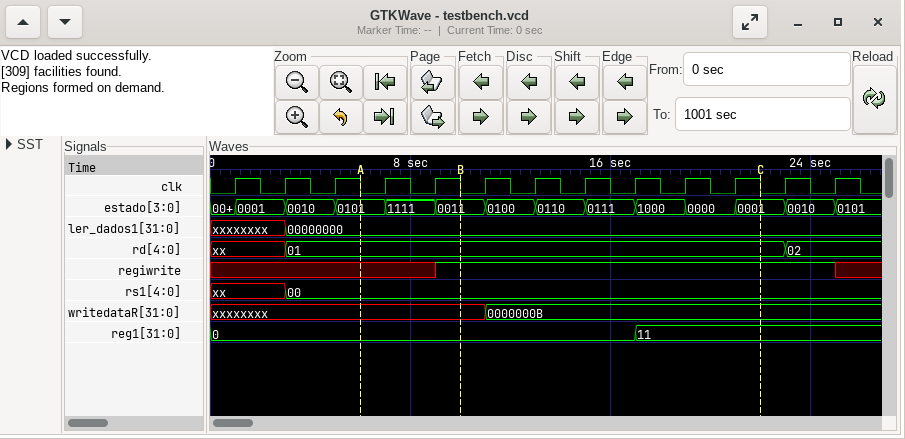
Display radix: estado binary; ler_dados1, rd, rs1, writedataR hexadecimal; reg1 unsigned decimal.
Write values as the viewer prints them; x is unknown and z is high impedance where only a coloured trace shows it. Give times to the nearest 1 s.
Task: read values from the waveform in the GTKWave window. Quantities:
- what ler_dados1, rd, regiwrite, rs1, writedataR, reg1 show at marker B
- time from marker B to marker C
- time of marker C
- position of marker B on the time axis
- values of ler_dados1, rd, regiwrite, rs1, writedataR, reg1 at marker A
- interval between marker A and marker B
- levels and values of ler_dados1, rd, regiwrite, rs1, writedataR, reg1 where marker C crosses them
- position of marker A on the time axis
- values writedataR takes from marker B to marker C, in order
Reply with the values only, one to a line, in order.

ler_dados1=00000000, rd=01, regiwrite=1, rs1=00, writedataR=xxxxxxxx, reg1=0
12 s
22 s
10 s
ler_dados1=00000000, rd=01, regiwrite=x, rs1=00, writedataR=xxxxxxxx, reg1=0
4 s
ler_dados1=00000000, rd=01, regiwrite=1, rs1=00, writedataR=0000000B, reg1=11
6 s
xxxxxxxx, 0000000B
